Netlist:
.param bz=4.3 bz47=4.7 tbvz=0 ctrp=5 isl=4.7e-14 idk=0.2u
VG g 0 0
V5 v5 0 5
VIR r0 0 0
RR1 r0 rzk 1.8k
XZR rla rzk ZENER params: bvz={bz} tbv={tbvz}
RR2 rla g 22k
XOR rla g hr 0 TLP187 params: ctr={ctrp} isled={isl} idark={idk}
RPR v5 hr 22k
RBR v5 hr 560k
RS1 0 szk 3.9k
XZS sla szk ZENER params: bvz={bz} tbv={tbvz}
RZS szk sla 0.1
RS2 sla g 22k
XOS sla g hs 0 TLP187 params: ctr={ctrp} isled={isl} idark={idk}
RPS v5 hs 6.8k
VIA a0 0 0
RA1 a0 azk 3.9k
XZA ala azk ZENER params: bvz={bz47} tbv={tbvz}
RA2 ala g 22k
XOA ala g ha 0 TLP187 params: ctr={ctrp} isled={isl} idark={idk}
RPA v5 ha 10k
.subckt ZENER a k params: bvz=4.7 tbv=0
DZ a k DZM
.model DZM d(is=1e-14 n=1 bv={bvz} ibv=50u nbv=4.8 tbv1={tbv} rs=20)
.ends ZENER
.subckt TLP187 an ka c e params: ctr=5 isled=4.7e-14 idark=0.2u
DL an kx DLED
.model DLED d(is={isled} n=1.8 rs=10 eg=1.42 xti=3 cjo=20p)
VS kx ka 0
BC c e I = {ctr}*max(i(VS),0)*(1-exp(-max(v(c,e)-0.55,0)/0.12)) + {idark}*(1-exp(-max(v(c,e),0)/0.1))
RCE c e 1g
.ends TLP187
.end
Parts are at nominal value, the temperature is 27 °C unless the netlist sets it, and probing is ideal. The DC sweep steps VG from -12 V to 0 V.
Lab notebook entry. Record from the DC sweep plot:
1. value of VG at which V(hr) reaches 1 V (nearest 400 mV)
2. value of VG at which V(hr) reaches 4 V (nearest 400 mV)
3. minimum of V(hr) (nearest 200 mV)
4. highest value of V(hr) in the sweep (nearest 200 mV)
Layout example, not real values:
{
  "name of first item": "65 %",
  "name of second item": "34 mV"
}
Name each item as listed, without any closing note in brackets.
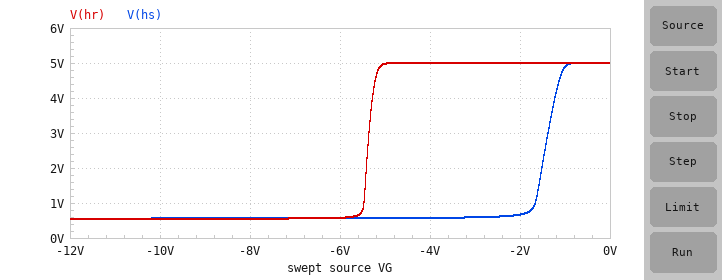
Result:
{
  "value of VG at which V(hr) reaches 1 V": "-5.6 V",
  "value of VG at which V(hr) reaches 4 V": "-5.2 V",
  "minimum of V(hr)": "600 mV",
  "highest value of V(hr) in the sweep": "5.0 V"
}
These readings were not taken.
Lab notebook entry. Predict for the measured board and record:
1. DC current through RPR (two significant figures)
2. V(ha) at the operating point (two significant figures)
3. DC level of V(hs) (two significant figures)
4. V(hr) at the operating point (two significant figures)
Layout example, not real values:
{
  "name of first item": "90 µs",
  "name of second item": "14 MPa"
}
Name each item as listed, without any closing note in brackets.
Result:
{
  "DC current through RPR": "200 nA",
  "V(ha) at the operating point": "5.0 V",
  "DC level of V(hs)": "5.0 V",
  "V(hr) at the operating point": "5.0 V"
}
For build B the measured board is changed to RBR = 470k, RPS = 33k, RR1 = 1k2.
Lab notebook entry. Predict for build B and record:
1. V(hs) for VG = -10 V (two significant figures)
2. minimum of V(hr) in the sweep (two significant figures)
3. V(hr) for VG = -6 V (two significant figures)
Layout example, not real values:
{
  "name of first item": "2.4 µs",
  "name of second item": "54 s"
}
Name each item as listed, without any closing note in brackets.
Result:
{
  "V(hs) for VG = -10 V": "550 mV",
  "minimum of V(hr) in the sweep": "550 mV",
  "V(hr) for VG = -6 V": "570 mV"
}
